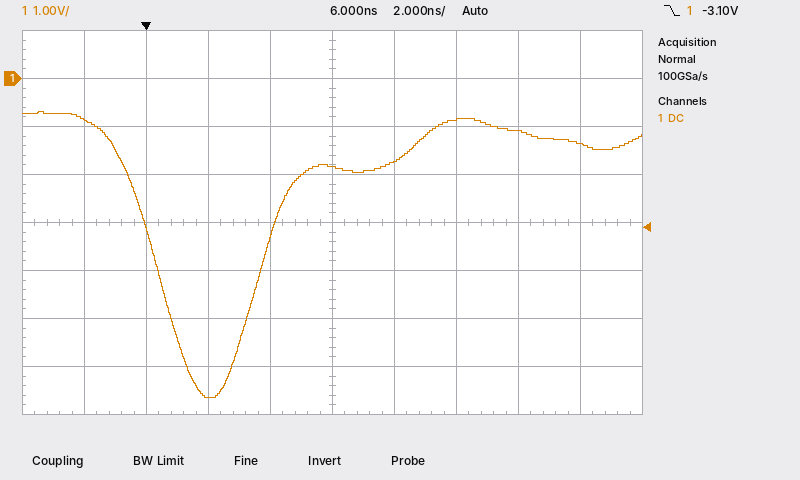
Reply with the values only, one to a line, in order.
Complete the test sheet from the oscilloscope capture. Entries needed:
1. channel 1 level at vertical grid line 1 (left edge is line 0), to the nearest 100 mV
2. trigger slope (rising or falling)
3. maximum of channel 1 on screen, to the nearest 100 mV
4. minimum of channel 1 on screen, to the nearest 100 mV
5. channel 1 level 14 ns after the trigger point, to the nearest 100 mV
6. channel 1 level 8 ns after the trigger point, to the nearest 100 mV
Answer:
-900 mV
falling
-700 mV
-6.6 V
-1.4 V
-1.7 V
